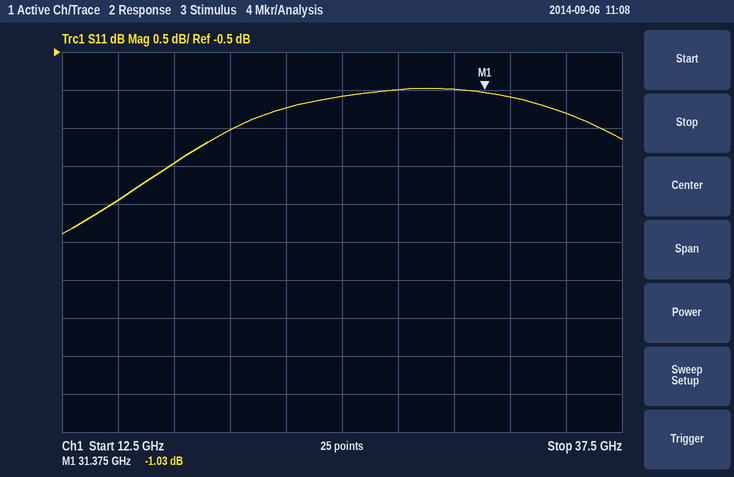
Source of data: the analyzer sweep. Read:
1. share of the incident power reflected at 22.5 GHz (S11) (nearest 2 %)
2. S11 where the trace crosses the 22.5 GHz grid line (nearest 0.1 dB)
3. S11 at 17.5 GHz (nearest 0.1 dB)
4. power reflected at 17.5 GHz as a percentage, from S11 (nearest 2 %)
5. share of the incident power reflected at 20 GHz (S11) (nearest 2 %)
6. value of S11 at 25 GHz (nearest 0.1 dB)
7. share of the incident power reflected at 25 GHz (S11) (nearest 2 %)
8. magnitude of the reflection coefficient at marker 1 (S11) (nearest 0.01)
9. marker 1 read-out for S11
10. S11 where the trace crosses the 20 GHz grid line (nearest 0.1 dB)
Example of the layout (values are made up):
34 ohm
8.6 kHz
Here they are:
76 %
-1.2 dB
-2.0 dB
64 %
70 %
-1.1 dB
78 %
0.89
-1.03 dB
-1.5 dB
